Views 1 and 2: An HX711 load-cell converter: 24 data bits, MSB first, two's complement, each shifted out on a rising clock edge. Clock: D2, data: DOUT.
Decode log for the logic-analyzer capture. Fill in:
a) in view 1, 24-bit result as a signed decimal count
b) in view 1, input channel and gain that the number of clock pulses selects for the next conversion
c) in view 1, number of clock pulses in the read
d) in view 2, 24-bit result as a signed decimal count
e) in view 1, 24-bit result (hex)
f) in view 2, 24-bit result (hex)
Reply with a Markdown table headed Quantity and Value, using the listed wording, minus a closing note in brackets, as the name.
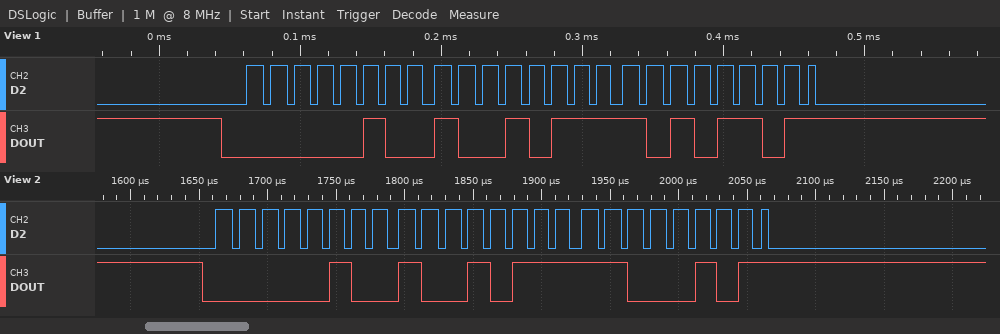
| Quantity | Value |
|---|---|
| in view 1, 24-bit result as a signed decimal count | 300973 |
| in view 1, input channel and gain that the number of clock pulses selects for the next conversion | channel A, gain 128 |
| in view 1, number of clock pulses in the read | 25 |
| in view 2, 24-bit result as a signed decimal count | 300997 |
| in view 1, 24-bit result | 0x0497AD |
| in view 2, 24-bit result | 0x0497C5 |
